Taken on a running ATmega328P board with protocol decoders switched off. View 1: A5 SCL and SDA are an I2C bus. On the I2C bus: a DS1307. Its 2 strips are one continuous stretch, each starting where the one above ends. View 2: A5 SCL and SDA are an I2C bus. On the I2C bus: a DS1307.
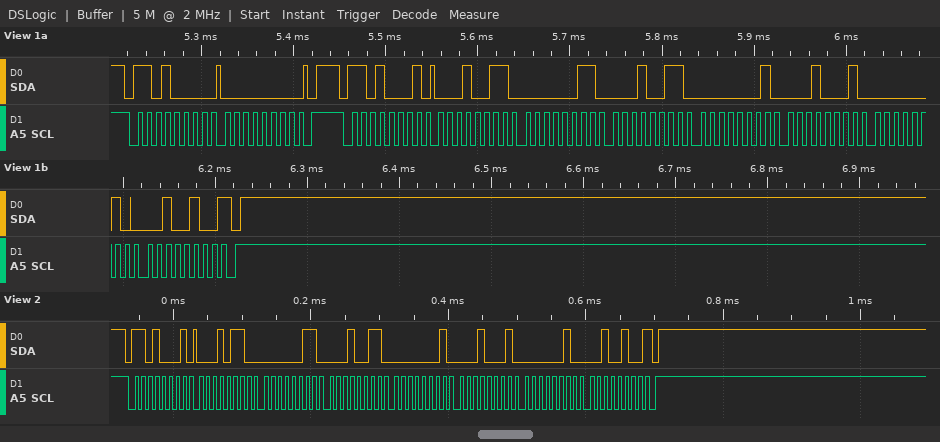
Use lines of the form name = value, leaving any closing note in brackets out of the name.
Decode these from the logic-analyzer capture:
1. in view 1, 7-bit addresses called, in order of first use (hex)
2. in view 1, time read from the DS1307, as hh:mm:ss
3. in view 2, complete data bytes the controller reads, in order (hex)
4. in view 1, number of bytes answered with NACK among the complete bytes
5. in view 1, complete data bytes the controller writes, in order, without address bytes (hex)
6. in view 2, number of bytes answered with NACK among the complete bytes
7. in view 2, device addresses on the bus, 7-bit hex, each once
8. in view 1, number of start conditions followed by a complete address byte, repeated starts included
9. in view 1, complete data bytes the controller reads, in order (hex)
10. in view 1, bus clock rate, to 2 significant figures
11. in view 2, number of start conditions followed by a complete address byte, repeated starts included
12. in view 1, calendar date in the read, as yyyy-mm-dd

in view 1, 7-bit addresses called, in order of first use = 0x68
in view 1, time read from the DS1307, as hh:mm:ss = 13:03:13
in view 2, complete data bytes the controller reads, in order = 16 03 13 01 11 02 24
in view 1, number of bytes answered with NACK among the complete bytes = 1
in view 1, complete data bytes the controller writes, in order, without address bytes = 00
in view 2, number of bytes answered with NACK among the complete bytes = 1
in view 2, device addresses on the bus, 7-bit hex, each once = 0x68
in view 1, number of start conditions followed by a complete address byte, repeated starts included = 2
in view 1, complete data bytes the controller reads, in order = 13 03 13 01 11 02 24
in view 1, bus clock rate, to 2 significant figures = 100 kHz
in view 2, number of start conditions followed by a complete address byte, repeated starts included = 1
in view 1, calendar date in the read, as yyyy-mm-dd = 2024-02-11
